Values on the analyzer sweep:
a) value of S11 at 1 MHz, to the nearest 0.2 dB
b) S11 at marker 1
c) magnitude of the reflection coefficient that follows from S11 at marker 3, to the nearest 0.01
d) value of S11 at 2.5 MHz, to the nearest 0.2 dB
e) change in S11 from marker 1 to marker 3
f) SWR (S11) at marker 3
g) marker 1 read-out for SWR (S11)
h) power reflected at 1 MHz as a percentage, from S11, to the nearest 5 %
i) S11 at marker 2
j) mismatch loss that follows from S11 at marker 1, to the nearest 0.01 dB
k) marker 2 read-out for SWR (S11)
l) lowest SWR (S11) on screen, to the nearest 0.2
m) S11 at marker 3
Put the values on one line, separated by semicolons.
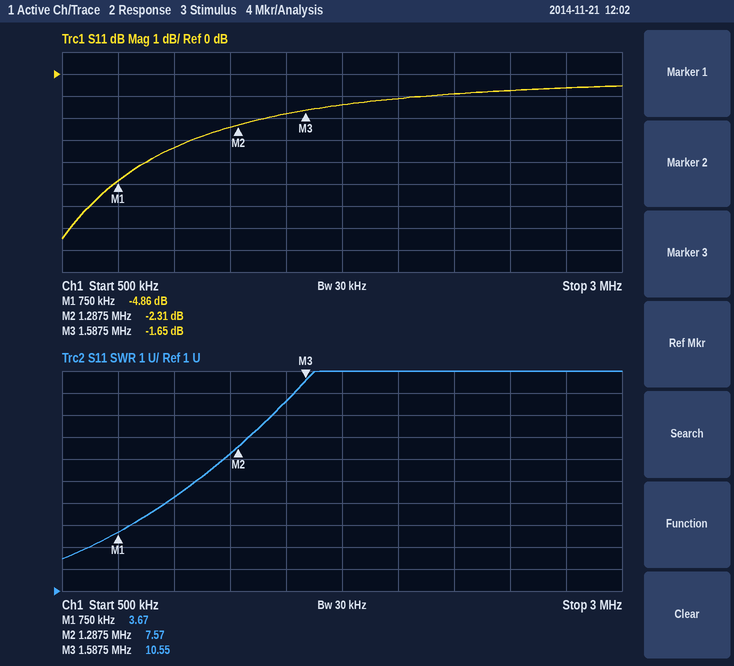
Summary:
-3.4 dB; -4.86 dB; 0.83; -0.8 dB; 3.21 dB; 10.55; 3.67; 45 %; -2.31 dB; 1.72 dB; 7.57; 2.4; -1.65 dB
